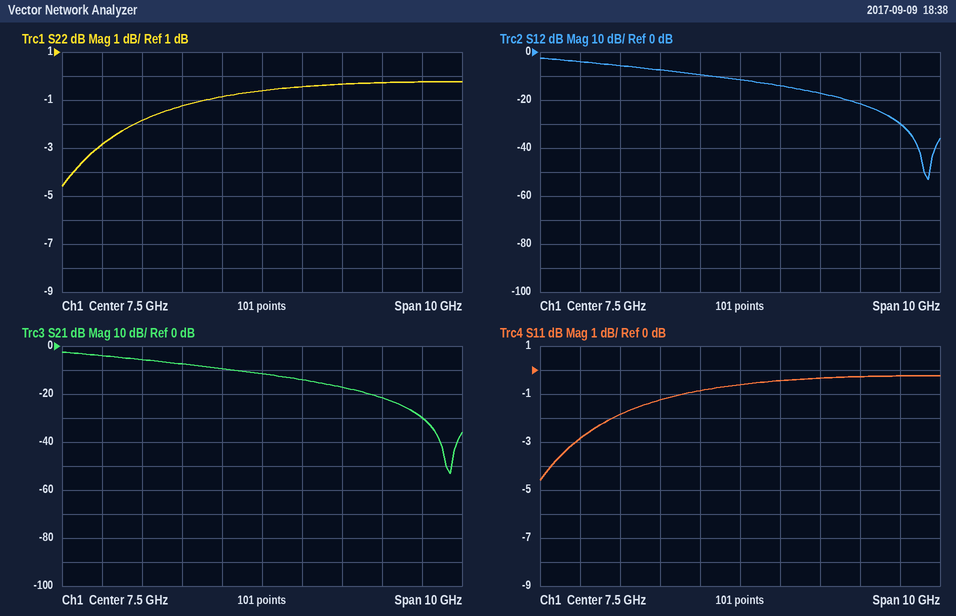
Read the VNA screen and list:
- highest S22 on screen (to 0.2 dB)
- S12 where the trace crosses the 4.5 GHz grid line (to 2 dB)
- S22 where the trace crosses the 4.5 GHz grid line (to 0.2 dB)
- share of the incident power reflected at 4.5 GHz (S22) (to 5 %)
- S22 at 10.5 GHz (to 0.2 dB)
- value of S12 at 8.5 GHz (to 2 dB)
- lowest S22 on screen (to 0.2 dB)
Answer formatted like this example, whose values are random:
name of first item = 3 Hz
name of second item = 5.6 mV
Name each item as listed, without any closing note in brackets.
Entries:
highest S22 on screen = -0.2 dB
S12 where the trace crosses the 4.5 GHz grid line = -6 dB
S22 where the trace crosses the 4.5 GHz grid line = -1.8 dB
share of the incident power reflected at 4.5 GHz (S22) = 65 %
S22 at 10.5 GHz = -0.2 dB
value of S12 at 8.5 GHz = -14 dB
lowest S22 on screen = -4.6 dB
